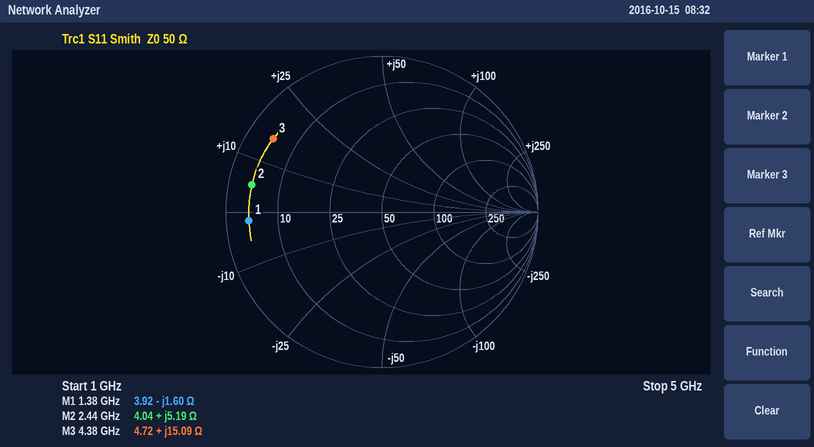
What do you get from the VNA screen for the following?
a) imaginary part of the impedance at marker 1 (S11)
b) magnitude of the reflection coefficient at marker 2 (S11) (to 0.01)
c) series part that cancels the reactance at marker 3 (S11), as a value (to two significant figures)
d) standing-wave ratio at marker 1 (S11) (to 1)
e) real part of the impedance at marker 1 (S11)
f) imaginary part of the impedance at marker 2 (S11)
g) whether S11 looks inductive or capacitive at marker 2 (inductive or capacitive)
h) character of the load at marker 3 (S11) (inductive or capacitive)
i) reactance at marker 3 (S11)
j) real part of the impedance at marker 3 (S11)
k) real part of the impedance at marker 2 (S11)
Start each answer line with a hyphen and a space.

- -1.60 Ω
- 0.85
- 2.4 pF
- 13
- 3.92 Ω
- +5.19 Ω
- inductive
- inductive
- +15.09 Ω
- 4.72 Ω
- 4.04 Ω
